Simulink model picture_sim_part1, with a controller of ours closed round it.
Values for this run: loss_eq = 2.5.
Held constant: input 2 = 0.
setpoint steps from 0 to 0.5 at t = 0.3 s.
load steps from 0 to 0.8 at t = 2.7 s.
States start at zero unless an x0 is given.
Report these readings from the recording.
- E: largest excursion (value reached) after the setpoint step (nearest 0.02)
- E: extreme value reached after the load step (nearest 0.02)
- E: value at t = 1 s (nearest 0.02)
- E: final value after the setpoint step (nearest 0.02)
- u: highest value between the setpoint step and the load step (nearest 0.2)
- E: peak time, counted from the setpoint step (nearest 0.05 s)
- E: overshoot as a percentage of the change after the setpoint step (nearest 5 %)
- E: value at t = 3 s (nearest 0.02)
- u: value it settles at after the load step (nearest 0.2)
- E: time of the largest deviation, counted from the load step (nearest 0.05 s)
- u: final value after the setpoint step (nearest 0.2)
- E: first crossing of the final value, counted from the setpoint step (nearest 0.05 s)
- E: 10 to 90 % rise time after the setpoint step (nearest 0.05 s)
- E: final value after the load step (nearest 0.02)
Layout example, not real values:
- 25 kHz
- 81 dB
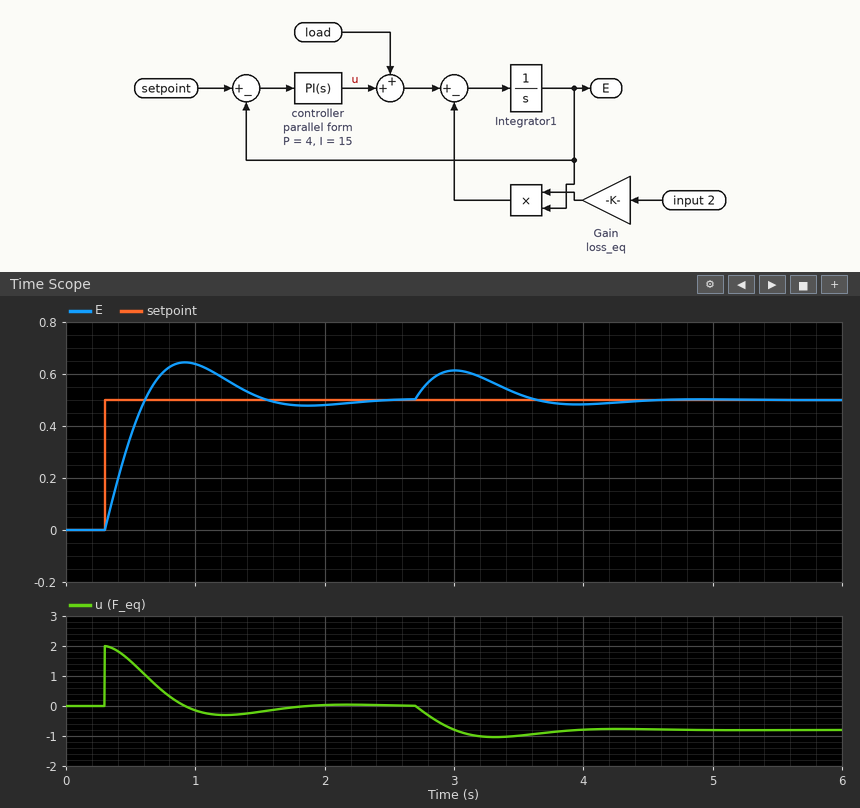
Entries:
- 0.64
- 0.62
- 0.64
- 0.50
- 2.0
- 0.60 s
- 30 %
- 0.62
- -0.8
- 0.30 s
- 0.0
- 0.30 s
- 0.25 s
- 0.50
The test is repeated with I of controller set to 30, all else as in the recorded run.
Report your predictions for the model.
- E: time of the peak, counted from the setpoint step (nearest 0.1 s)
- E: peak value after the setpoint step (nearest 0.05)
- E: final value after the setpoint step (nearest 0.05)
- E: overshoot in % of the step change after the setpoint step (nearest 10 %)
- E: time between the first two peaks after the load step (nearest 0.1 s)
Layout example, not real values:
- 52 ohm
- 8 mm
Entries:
- 0.5 s
- 0.70
- 0.50
- 40 %
- 1.2 s
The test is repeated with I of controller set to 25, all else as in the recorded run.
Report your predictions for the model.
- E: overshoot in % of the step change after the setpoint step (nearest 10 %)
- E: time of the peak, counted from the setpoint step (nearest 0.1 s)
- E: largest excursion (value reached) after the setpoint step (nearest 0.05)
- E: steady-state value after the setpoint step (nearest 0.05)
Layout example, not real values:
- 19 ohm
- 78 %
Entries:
- 40 %
- 0.5 s
- 0.70
- 0.50
